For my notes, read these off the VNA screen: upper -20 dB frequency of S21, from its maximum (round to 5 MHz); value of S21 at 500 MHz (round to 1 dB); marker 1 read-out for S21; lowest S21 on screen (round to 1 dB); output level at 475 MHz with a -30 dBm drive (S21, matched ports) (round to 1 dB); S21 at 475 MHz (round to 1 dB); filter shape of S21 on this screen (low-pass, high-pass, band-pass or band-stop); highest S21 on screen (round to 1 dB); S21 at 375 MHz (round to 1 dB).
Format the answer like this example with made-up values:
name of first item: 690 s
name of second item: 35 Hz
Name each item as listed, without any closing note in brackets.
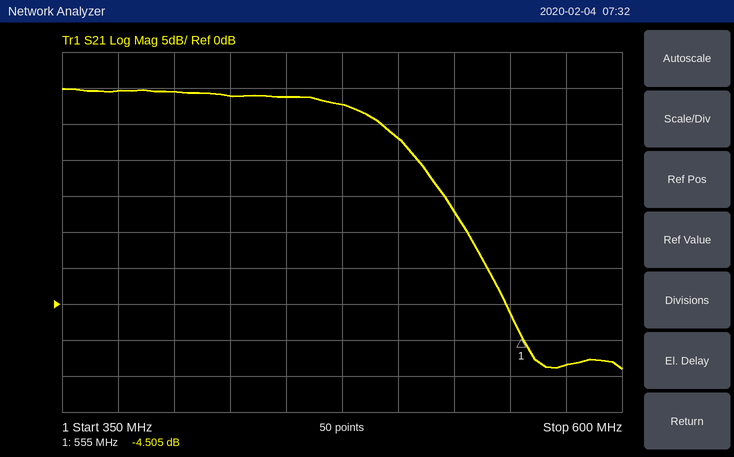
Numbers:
upper -20 dB frequency of S21, from its maximum: 530 MHz
value of S21 at 500 MHz: 23 dB
marker 1 read-out for S21: -4.505 dB
lowest S21 on screen: -9 dB
output level at 475 MHz with a -30 dBm drive (S21, matched ports): -2 dBm
S21 at 475 MHz: 28 dB
filter shape of S21 on this screen: low-pass
highest S21 on screen: 30 dB
S21 at 375 MHz: 30 dB
